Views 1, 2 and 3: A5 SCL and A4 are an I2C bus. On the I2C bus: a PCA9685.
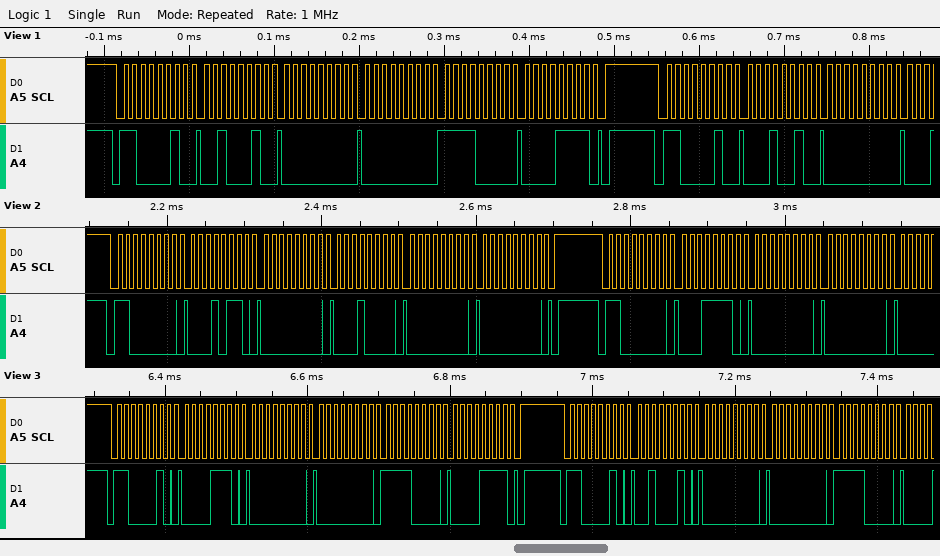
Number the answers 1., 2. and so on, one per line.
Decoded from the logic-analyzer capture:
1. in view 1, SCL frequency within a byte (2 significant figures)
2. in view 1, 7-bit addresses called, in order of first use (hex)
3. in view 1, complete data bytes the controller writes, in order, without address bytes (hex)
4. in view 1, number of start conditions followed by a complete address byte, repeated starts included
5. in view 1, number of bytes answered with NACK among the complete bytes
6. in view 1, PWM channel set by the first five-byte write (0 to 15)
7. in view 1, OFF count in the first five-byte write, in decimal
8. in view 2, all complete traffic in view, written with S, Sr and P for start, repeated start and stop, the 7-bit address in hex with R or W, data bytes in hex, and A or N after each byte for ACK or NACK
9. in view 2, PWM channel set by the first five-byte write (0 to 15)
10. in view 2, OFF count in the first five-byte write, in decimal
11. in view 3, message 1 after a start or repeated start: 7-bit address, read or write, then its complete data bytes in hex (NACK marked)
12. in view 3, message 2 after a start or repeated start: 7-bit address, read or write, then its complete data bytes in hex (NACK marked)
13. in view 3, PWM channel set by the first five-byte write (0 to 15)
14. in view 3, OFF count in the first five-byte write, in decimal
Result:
1. 100 kHz
2. 0x61
3. 22 00 00 F0 0F 12 00
4. 2
5. 0
6. 7
7. 4080
8. S 60W A 16 A 00 A 10 A 00 A 00 A P S 60W A 1E A 00 A 00 A
9. 4
10. 0
11. 0x61 write: 0E 00 00 F0 0F
12. 0x61 write: 22 00 00 F0
13. 2
14. 4080
